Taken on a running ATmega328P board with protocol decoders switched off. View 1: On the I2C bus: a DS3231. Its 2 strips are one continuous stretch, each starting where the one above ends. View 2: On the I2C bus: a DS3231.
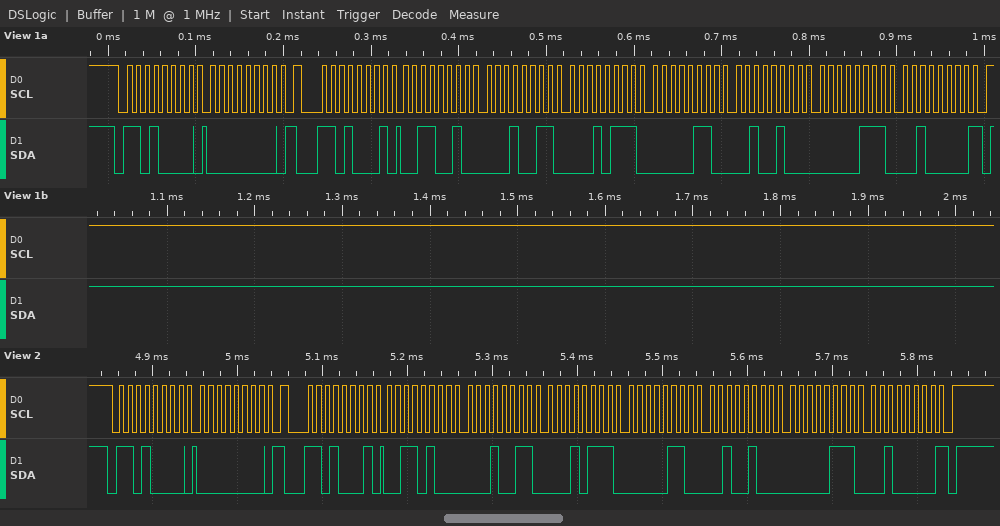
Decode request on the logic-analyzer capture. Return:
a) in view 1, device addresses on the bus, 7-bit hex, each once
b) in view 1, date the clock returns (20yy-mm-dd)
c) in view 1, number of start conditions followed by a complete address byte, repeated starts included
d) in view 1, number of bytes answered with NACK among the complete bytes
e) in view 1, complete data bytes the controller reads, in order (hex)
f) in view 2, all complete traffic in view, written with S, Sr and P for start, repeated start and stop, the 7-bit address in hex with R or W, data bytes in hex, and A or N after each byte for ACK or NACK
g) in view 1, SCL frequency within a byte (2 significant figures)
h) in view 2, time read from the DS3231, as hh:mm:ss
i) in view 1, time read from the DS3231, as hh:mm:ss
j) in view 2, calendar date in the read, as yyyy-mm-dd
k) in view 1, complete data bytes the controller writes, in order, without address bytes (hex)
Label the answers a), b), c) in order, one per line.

a) 0x68
b) 2020-07-24
c) 2
d) 1
e) 32 13 17 06 24 07 20
f) S 68W A 00 A Sr 68R A 34 A 13 A 17 A 06 A 24 A 07 A 20 N P
g) 100 kHz
h) 17:13:34
i) 17:13:32
j) 2020-07-24
k) 00
